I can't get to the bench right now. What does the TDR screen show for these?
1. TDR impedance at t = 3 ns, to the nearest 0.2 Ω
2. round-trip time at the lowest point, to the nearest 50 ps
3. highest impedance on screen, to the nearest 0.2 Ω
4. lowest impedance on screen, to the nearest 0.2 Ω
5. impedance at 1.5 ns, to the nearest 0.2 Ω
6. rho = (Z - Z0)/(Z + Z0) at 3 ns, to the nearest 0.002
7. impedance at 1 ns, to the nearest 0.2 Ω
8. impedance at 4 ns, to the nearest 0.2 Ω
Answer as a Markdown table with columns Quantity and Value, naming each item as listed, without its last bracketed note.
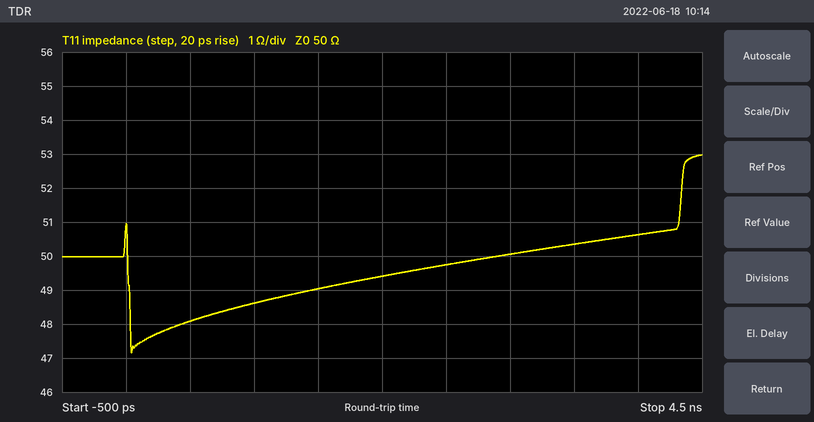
| Quantity | Value |
|---|---|
| TDR impedance at t = 3 ns, to the nearest 0.2 Ω | 50.0 Ω |
| round-trip time at the lowest point, to the nearest 50 ps | 50 ps |
| highest impedance on screen, to the nearest 0.2 Ω | 53.0 Ω |
| lowest impedance on screen, to the nearest 0.2 Ω | 47.2 Ω |
| impedance at 1.5 ns, to the nearest 0.2 Ω | 49.0 Ω |
| rho = (Z - Z0)/(Z + Z0) at 3 ns, to the nearest 0.002 | 0.000 |
| impedance at 1 ns, to the nearest 0.2 Ω | 48.6 Ω |
| impedance at 4 ns, to the nearest 0.2 Ω | 50.6 Ω |
